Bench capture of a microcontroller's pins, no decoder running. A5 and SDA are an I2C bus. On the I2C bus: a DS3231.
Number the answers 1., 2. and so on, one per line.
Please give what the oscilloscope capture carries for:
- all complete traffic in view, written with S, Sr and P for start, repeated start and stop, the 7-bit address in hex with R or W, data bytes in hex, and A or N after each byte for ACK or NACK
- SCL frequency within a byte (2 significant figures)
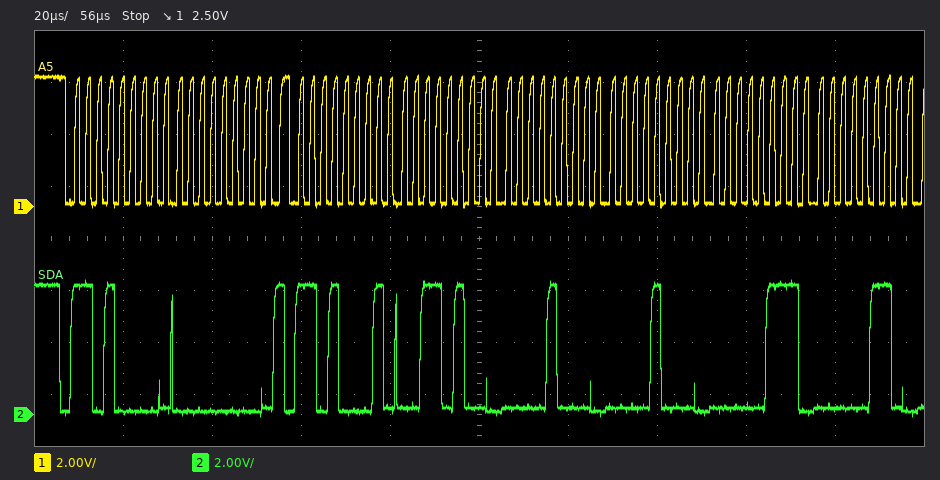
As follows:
1. S 68W A 00 A Sr 68R A 34 A 08 A 08 A 07 A 06 A
2. 400 kHz
